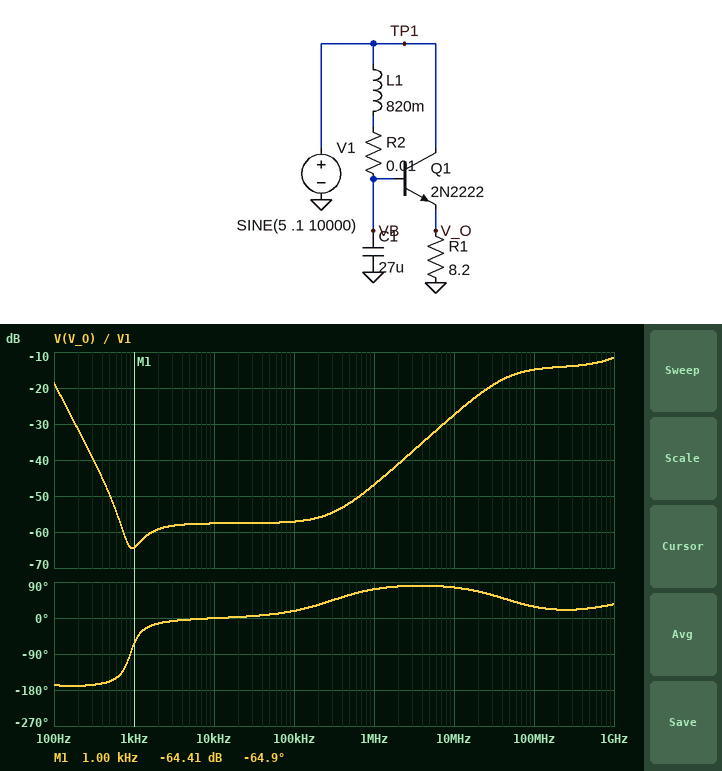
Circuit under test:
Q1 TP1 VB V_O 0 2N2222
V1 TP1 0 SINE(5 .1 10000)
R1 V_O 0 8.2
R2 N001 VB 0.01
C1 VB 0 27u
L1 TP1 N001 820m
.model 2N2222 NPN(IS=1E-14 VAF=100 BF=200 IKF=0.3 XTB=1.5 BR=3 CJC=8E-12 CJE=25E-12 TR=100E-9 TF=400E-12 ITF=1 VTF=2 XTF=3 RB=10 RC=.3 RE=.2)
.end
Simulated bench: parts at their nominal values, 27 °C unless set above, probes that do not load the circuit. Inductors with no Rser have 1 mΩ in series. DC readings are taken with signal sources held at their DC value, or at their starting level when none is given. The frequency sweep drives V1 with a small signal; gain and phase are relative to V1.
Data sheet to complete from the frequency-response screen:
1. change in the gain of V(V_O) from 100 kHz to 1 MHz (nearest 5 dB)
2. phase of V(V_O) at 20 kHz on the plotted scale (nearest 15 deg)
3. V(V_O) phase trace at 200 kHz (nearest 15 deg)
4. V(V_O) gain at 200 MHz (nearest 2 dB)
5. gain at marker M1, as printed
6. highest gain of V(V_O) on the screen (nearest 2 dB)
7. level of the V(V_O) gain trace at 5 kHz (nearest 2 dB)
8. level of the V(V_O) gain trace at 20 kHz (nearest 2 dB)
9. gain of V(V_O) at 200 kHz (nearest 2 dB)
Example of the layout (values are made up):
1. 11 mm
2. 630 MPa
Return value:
1. 10 dB
2. 0 deg
3. 30 deg
4. -14 dB
5. -64.41 dB
6. -12 dB
7. -58 dB
8. -58 dB
9. -56 dB
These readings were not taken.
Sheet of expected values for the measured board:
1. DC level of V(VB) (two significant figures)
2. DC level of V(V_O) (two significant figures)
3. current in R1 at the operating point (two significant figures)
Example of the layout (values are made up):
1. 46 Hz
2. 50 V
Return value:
1. 5.0 V
2. 4.0 V
3. 490 mA
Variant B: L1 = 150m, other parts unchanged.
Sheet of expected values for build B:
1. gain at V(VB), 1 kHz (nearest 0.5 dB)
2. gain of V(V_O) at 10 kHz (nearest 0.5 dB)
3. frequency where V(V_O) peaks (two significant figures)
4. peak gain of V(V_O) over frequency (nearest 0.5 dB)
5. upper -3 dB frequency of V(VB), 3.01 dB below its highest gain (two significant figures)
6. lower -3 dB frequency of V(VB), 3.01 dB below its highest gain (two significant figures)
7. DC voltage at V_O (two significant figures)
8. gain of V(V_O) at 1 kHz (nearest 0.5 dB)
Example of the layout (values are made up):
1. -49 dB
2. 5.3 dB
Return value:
1. -44.0 dB
2. -58.0 dB
3. 78 Hz
4. 14.0 dB
5. 85 Hz
6. 71 Hz
7. 4.0 V
8. -46.5 dB
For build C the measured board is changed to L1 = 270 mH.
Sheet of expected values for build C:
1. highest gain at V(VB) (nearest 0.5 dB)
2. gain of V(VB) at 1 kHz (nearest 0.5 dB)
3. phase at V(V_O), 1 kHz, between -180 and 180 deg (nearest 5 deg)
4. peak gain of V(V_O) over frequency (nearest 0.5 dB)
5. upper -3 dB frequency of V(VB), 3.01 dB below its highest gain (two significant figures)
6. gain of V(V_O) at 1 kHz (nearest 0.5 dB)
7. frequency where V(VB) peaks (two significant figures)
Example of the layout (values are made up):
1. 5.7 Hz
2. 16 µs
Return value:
1. 12.0 dB
2. -49.0 dB
3. -165 deg
4. 11.5 dB
5. 65 Hz
6. -54.0 dB
7. 58 Hz
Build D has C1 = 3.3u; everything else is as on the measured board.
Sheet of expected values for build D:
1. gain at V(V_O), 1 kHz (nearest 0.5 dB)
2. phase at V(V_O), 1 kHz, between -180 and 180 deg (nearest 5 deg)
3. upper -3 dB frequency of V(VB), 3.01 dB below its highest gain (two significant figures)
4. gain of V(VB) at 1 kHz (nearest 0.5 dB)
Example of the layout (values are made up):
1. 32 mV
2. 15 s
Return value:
1. -41.0 dB
2. -140 deg
3. 110 Hz
4. -39.5 dB
